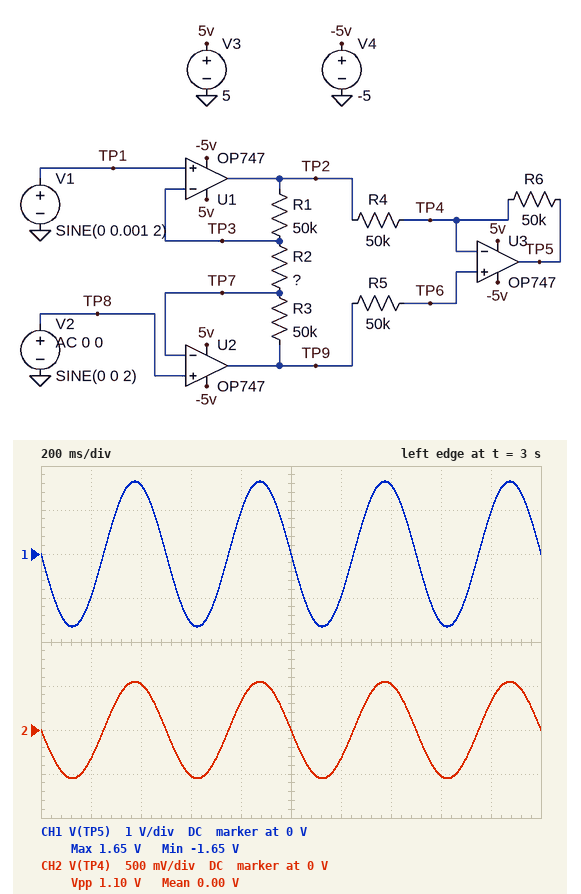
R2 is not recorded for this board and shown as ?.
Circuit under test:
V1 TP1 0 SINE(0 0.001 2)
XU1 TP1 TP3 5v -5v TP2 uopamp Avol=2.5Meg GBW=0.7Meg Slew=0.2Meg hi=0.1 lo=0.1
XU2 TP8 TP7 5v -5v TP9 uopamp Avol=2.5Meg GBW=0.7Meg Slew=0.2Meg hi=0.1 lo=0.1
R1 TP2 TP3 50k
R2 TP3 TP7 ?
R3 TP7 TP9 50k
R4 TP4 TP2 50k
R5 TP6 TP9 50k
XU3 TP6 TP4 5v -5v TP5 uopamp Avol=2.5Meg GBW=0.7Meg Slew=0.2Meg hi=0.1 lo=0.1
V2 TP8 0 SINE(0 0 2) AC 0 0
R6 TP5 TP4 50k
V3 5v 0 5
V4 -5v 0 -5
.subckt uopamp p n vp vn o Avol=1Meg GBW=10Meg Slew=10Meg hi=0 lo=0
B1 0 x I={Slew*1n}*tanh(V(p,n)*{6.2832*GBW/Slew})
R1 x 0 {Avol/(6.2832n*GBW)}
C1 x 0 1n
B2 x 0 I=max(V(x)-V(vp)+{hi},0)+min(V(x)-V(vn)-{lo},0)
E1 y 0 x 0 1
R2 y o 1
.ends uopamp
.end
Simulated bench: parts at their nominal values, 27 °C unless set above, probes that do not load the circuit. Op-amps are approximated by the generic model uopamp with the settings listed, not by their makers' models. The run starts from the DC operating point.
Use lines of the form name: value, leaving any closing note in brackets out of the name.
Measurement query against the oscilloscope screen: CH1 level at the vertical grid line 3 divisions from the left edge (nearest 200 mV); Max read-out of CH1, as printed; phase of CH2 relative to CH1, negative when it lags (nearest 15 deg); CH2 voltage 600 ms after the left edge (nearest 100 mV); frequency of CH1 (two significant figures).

CH1 level at the vertical grid line 3 divisions from the left edge: -1.6 V
Max read-out of CH1, as printed: 1.65 V
phase of CH2 relative to CH1, negative when it lags: 0 deg
CH2 voltage 600 ms after the left edge: -500 mV
frequency of CH1: 2.0 Hz
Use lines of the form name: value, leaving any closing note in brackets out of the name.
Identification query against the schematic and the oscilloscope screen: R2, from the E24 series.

R2, from the E24 series: 91 Ω
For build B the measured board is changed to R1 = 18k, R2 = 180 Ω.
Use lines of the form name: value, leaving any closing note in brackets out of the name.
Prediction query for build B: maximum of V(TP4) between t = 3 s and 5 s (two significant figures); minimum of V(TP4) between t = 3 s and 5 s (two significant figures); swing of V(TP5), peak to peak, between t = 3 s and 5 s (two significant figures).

maximum of V(TP4) between t = 3 s and 5 s: 280 mV
minimum of V(TP4) between t = 3 s and 5 s: -280 mV
swing of V(TP5), peak to peak, between t = 3 s and 5 s: 1.3 V
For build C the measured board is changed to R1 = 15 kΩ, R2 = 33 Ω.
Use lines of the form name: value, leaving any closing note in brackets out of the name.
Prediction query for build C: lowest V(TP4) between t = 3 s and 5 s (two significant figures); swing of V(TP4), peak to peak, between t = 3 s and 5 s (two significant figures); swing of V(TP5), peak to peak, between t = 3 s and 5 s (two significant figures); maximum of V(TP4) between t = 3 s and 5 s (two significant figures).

lowest V(TP4) between t = 3 s and 5 s: -1.5 V
swing of V(TP4), peak to peak, between t = 3 s and 5 s: 3.0 V
swing of V(TP5), peak to peak, between t = 3 s and 5 s: 7.0 V
maximum of V(TP4) between t = 3 s and 5 s: 1.5 V
